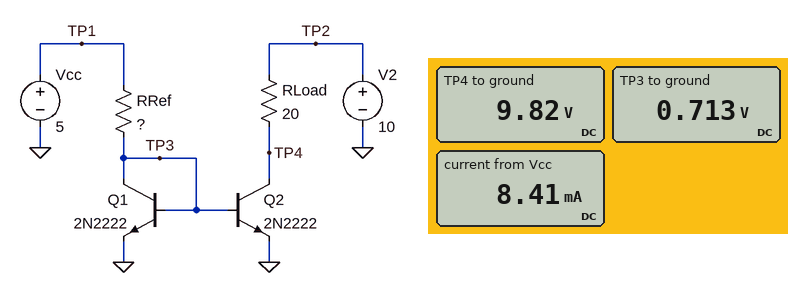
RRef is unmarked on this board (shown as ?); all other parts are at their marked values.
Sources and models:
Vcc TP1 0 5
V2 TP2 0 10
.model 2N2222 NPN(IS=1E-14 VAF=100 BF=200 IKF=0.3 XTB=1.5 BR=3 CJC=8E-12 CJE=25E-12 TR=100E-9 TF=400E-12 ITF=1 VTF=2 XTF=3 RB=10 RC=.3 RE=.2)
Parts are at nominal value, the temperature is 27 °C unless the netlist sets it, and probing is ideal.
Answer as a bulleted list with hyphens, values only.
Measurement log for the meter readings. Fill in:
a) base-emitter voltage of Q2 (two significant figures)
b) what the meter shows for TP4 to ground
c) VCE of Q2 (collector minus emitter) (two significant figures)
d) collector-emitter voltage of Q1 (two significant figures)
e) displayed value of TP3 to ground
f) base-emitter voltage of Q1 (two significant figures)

- 710 mV
- 9.82 V
- 9.8 V
- 710 mV
- 0.713 V
- 710 mV
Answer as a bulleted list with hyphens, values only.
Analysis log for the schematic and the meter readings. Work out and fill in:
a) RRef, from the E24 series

- 510 Ω
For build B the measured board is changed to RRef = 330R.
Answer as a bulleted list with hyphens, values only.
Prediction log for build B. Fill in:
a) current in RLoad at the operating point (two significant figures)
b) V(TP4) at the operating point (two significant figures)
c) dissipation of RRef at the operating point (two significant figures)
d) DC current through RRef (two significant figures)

- 14 mA
- 9.7 V
- 55 mW
- 13 mA
